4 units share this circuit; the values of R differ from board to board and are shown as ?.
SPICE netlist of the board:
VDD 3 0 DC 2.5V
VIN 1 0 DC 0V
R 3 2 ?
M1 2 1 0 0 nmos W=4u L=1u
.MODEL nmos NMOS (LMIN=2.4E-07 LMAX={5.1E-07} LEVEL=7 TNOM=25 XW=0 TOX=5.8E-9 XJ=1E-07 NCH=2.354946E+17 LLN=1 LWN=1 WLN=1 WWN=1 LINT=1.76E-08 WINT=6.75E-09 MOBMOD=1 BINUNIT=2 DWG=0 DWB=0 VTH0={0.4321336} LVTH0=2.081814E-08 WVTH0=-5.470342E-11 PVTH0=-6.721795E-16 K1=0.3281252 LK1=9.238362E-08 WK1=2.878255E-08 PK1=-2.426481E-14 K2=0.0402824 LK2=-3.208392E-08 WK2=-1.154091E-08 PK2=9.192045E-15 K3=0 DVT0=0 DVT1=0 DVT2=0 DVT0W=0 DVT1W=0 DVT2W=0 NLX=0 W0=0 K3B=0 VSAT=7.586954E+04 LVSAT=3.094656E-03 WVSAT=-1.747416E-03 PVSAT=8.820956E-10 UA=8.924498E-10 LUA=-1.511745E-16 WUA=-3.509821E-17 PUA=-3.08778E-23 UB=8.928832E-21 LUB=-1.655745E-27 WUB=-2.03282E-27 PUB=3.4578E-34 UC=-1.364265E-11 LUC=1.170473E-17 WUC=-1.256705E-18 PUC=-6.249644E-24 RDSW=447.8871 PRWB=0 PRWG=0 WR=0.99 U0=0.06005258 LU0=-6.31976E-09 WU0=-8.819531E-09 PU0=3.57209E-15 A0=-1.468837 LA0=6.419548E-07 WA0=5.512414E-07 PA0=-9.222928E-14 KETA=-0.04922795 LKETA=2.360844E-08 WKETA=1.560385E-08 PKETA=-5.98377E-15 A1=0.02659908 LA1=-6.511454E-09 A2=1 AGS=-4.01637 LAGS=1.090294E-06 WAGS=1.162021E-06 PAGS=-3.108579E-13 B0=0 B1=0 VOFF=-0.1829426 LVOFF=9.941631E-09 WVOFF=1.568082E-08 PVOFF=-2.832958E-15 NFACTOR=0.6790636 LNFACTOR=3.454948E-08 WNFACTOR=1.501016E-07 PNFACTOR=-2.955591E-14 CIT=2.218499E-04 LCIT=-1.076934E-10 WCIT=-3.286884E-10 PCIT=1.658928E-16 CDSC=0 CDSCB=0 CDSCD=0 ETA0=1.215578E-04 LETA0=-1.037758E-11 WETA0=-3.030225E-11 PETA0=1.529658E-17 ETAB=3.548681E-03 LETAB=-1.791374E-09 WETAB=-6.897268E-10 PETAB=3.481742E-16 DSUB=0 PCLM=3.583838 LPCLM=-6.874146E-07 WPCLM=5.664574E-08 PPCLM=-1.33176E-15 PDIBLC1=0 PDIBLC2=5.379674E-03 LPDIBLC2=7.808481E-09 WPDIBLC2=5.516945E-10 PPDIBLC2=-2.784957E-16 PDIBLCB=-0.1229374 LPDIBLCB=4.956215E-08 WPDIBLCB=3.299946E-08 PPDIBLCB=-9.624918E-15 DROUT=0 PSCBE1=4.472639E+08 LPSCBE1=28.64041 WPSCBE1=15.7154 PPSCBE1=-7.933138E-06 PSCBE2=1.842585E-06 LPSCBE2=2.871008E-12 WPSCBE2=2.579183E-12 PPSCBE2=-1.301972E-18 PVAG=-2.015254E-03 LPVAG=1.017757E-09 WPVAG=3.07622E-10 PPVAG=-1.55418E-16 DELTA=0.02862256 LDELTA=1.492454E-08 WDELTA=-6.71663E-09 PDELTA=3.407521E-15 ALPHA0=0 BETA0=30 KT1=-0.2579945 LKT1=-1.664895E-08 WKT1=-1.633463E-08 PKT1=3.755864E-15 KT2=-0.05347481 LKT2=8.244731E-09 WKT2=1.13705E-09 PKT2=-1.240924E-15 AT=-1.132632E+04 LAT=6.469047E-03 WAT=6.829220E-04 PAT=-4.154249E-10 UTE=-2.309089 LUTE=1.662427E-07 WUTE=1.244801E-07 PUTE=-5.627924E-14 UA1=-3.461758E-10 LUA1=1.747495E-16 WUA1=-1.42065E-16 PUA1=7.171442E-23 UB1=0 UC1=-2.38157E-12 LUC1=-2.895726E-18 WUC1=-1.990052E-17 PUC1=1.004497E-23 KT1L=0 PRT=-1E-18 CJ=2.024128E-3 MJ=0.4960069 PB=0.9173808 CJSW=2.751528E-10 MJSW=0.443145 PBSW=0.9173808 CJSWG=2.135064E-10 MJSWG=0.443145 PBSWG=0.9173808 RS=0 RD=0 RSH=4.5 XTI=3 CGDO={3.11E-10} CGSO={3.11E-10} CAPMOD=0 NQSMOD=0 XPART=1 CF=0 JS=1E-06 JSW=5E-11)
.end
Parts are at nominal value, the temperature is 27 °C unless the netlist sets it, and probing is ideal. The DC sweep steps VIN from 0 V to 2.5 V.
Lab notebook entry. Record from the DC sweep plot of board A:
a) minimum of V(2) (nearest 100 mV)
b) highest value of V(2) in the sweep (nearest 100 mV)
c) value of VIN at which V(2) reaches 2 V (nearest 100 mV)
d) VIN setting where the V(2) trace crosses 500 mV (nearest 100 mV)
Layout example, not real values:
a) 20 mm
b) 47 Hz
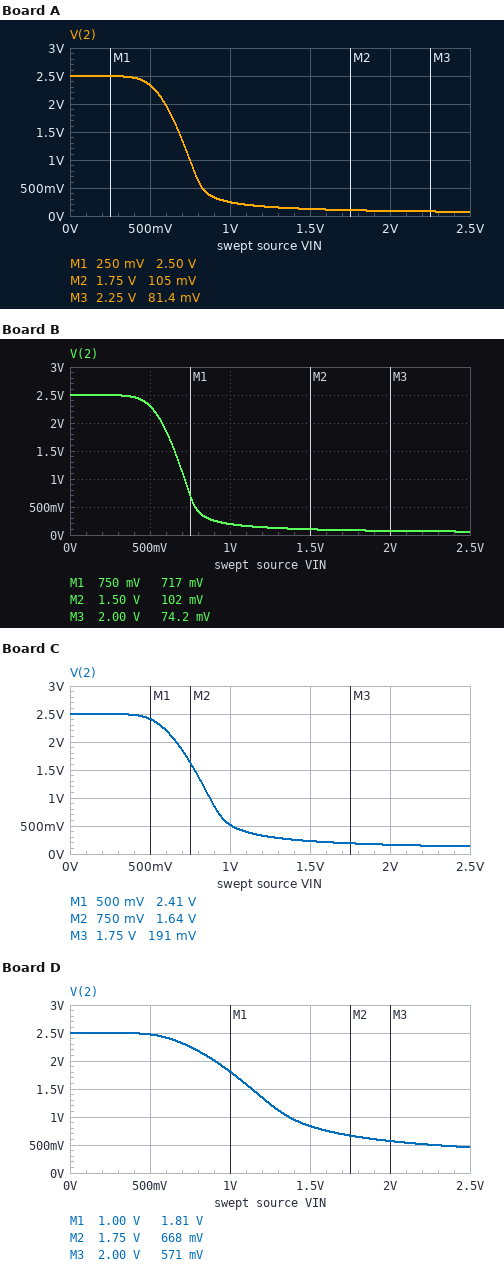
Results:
a) 100 mV
b) 2.5 V
c) 600 mV
d) 800 mV
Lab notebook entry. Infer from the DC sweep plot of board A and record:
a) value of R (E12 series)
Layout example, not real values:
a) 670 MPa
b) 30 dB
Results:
a) 22 kΩ
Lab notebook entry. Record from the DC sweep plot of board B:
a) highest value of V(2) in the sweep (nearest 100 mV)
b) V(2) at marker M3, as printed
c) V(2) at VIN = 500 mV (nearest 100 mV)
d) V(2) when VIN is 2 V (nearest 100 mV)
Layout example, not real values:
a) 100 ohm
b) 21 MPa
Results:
a) 2.5 V
b) 74.2 mV
c) 2.3 V
d) 100 mV
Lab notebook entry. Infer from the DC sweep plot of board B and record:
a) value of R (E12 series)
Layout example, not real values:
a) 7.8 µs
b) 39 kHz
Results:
a) 27 kΩ
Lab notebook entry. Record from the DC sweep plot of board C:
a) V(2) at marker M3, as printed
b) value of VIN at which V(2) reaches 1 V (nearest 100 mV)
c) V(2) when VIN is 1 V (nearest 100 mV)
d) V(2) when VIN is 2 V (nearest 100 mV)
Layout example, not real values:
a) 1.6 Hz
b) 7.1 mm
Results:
a) 191 mV
b) 900 mV
c) 500 mV
d) 200 mV
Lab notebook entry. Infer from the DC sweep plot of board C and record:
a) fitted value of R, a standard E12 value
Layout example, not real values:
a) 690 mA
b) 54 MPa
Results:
a) 12 kΩ
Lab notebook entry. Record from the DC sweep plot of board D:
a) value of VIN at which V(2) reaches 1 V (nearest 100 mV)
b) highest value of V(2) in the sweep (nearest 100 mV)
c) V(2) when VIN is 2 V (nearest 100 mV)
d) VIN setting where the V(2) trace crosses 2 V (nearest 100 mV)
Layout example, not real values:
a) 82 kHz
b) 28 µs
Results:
a) 1.4 V
b) 2.5 V
c) 600 mV
d) 900 mV
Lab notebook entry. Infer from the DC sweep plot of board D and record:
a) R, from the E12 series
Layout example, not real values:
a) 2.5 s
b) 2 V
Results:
a) 3.3 kΩ
